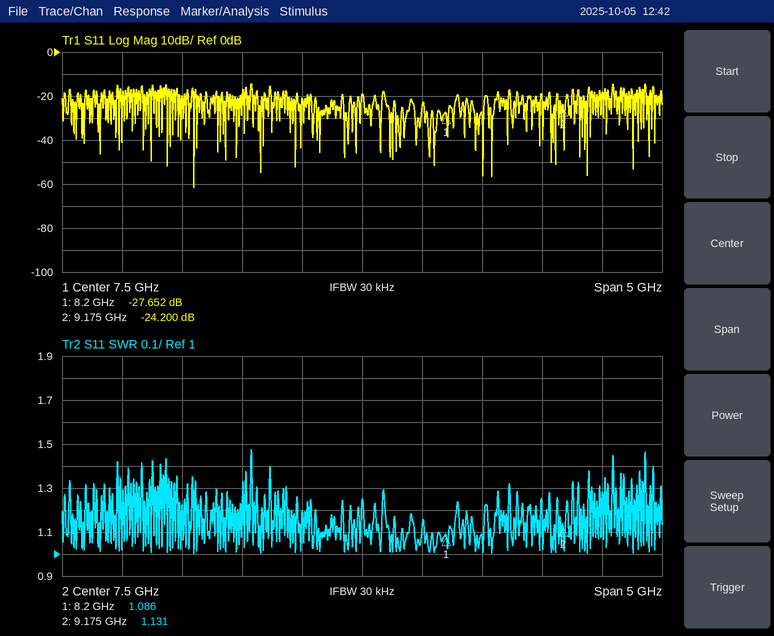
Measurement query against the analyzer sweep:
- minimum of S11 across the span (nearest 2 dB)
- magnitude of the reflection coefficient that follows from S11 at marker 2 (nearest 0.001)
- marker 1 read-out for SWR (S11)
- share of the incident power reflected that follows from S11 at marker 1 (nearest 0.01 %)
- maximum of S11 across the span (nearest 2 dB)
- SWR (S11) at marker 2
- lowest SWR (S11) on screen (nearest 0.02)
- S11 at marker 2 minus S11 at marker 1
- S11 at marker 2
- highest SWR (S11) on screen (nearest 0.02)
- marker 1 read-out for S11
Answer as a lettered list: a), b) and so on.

a) -62 dB
b) 0.062
c) 1.086
d) 0.17 %
e) -14 dB
f) 1.131
g) 1.00
h) 3.452 dB
i) -24.200 dB
j) 1.48
k) -27.652 dB
